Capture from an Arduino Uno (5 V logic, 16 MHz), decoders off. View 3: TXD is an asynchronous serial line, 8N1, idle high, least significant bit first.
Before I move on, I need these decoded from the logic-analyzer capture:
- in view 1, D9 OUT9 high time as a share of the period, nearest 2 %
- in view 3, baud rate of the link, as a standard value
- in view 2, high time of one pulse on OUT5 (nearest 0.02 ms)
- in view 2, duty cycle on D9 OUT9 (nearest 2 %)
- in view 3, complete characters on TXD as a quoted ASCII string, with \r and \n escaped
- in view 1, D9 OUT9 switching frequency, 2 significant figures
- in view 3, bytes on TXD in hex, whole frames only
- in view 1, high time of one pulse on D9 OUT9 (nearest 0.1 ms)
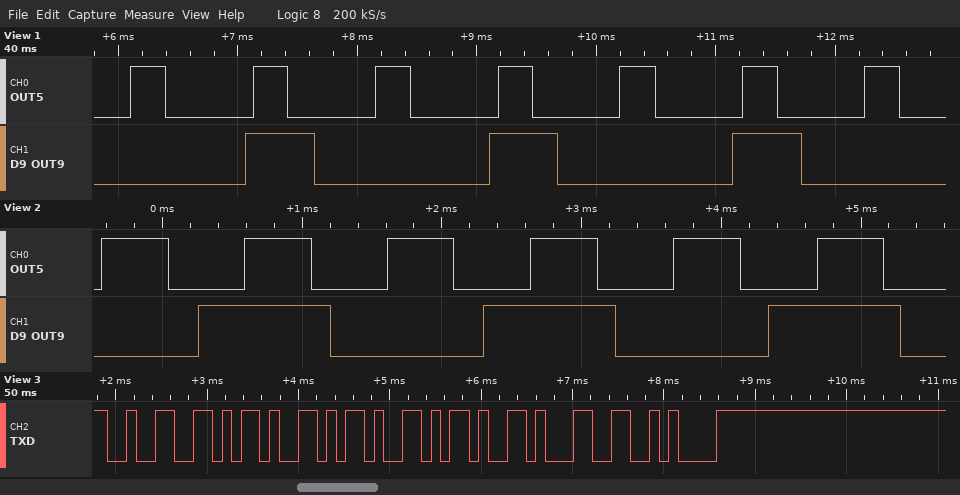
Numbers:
28 %
9600 baud
0.48 ms
46 %
"2---1\n"
490 Hz
0x32 0x2D 0x2D 0x2D 0x31 0x0A
0.6 ms
